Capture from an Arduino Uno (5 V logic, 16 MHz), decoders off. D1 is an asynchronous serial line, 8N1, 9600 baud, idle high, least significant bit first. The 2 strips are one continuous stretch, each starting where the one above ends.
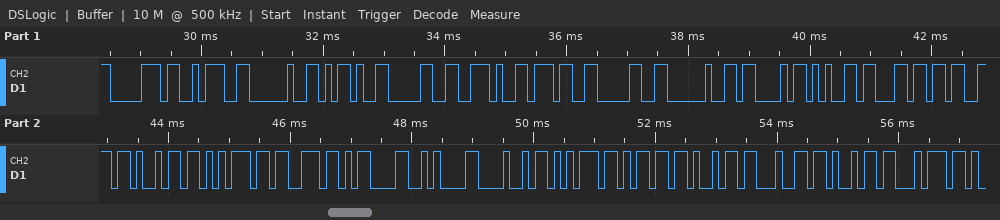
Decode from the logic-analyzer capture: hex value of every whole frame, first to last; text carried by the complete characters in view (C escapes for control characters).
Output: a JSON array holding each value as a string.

["0x70 0x3A 0x20 0x2D 0x30 0x2E 0x37 0x30 0x20 0x43 0x65 0x6C 0x73 0x69 0x75 0x73 0x0D 0x0A 0x48 0x75 0x6D 0x69 0x64 0x69 0x74", "\"p: -0.70 Celsius\\r\\nHumidit\""]
